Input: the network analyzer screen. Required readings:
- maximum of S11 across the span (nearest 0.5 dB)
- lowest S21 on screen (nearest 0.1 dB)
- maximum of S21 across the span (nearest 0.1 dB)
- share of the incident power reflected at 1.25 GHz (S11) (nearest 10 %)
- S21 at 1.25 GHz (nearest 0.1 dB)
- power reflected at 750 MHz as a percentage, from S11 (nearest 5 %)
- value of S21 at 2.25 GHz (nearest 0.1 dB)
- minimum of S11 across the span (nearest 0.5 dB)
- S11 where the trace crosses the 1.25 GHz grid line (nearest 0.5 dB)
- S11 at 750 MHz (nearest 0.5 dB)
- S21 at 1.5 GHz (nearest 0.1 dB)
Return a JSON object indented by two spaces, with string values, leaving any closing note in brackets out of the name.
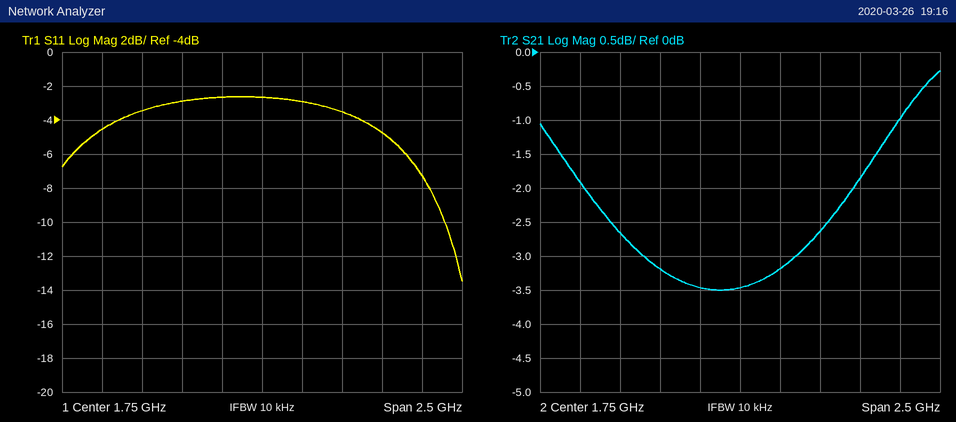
{
  "maximum of S11 across the span": "-2.5 dB",
  "lowest S21 on screen": "-3.5 dB",
  "maximum of S21 across the span": "-0.3 dB",
  "share of the incident power reflected at 1.25 GHz (S11)": "50 %",
  "S21 at 1.25 GHz": "-3.2 dB",
  "power reflected at 750 MHz as a percentage, from S11": "35 %",
  "value of S21 at 2.25 GHz": "-2.6 dB",
  "minimum of S11 across the span": "-13.5 dB",
  "S11 where the trace crosses the 1.25 GHz grid line": "-3.0 dB",
  "S11 at 750 MHz": "-4.5 dB",
  "S21 at 1.5 GHz": "-3.5 dB"
}
